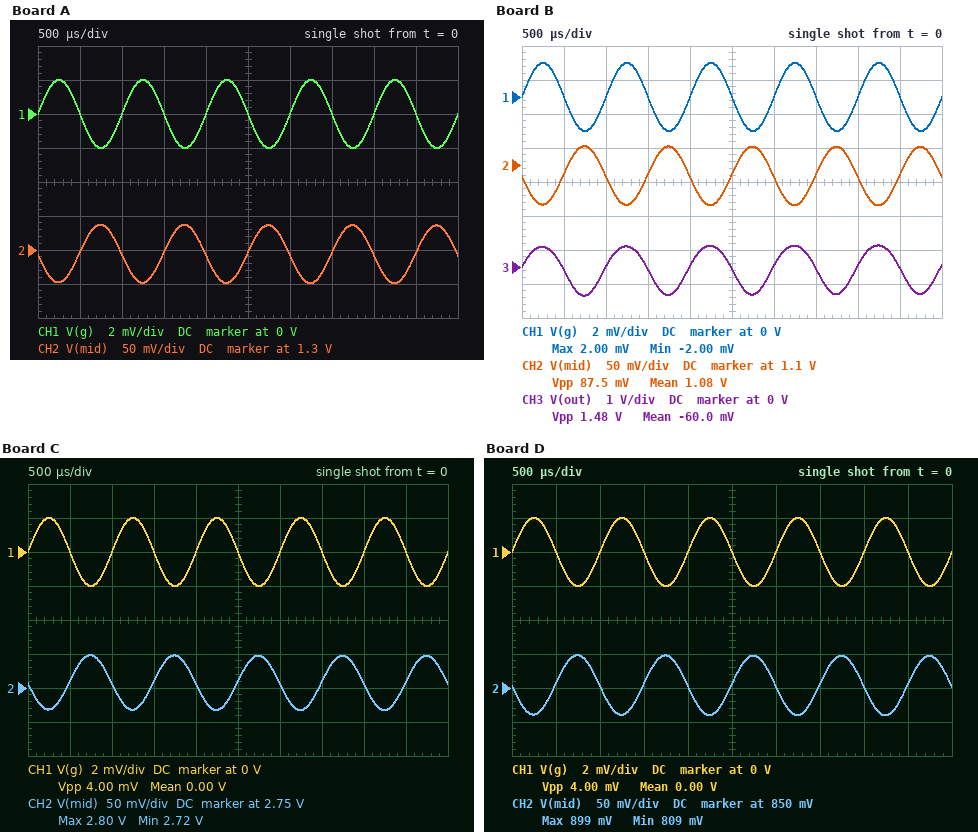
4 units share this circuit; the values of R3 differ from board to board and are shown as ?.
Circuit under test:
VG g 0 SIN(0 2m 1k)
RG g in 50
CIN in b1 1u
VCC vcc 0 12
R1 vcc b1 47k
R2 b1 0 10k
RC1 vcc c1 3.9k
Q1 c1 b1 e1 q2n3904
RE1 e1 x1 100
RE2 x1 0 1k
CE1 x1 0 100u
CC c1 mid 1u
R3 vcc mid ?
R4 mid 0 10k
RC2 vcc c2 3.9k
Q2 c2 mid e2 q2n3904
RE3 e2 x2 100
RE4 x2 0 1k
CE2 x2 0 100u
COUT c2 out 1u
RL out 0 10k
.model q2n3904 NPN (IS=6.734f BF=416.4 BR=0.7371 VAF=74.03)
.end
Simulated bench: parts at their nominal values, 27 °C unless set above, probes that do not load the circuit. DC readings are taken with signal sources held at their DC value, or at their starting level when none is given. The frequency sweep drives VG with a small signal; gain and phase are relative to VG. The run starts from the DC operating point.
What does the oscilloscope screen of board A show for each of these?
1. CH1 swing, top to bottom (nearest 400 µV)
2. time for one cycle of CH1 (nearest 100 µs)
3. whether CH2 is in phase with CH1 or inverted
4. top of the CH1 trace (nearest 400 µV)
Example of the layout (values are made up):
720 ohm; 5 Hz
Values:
4.0 mV; 1.0 ms; inverted; 2.0 mV
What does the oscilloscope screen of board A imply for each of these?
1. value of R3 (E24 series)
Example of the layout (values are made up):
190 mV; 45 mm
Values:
82 kΩ
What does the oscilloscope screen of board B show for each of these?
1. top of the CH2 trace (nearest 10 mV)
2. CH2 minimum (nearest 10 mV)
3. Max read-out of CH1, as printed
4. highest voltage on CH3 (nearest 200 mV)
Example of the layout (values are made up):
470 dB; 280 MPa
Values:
1.13 V; 1.04 V; 2.00 mV; 600 mV
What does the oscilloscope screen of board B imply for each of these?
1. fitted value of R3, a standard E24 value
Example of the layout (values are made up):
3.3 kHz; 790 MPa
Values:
100 kΩ
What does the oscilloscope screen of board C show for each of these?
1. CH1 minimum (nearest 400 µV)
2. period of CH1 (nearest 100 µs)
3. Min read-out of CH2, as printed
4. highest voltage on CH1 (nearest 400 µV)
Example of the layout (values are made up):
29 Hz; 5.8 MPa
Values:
-2.0 mV; 1.0 ms; 2.72 V; 2.0 mV
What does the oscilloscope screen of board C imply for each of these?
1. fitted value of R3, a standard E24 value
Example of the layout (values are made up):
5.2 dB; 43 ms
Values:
33 kΩ
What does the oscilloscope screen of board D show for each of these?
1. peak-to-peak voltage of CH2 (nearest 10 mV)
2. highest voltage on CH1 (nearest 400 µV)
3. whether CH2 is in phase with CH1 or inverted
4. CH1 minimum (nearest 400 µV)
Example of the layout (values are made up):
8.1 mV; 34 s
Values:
90 mV; 2.0 mV; inverted; -2.0 mV
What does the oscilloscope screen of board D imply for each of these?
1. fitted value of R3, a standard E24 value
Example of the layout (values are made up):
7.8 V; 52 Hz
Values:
130 kΩ
